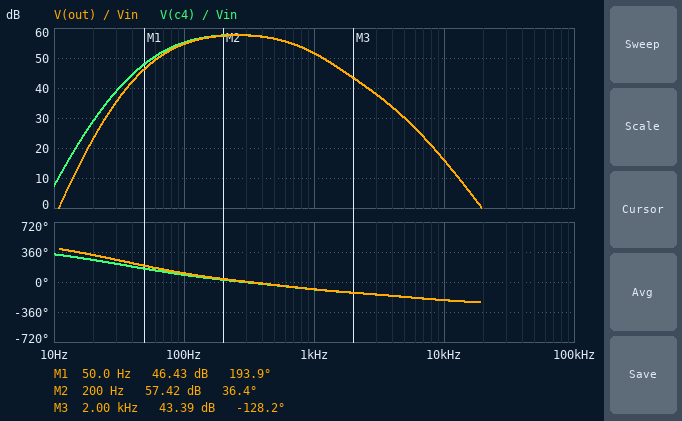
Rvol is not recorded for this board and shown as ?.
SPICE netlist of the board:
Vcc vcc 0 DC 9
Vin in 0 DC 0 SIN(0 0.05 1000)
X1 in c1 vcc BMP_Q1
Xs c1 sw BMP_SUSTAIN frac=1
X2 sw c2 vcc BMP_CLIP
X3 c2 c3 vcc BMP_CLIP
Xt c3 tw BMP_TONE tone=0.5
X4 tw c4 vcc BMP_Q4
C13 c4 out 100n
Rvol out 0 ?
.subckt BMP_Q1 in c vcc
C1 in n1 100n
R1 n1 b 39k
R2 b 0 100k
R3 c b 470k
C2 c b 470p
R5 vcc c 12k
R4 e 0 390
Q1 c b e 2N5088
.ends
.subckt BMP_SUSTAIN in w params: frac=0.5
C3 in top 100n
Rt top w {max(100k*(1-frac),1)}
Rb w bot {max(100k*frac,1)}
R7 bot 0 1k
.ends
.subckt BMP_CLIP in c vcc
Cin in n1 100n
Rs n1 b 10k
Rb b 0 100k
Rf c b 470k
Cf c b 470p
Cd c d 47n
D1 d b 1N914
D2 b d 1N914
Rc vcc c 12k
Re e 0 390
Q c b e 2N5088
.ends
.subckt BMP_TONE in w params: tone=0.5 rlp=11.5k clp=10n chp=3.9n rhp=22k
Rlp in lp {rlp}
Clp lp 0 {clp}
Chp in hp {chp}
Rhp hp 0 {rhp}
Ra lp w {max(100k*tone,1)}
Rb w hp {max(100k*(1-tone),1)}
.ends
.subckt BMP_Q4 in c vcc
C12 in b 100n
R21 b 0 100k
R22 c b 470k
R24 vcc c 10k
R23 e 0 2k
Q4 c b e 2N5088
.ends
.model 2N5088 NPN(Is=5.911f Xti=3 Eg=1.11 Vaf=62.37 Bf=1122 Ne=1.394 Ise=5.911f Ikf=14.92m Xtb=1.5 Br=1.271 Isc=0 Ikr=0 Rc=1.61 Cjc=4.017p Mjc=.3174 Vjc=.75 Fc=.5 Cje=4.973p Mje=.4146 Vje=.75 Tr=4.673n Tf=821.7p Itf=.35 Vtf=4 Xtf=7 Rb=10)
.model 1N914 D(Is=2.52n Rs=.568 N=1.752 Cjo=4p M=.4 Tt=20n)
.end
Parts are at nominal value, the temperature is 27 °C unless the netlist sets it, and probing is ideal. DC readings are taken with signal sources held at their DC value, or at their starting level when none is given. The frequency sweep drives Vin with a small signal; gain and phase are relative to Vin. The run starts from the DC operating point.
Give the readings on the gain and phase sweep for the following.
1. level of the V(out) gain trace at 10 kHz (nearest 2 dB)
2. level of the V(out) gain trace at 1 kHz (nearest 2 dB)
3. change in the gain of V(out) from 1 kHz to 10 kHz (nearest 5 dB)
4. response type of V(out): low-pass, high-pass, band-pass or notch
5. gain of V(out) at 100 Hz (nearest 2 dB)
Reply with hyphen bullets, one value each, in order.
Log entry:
- 16 dB
- 52 dB
- -35 dB
- band-pass
- 54 dB
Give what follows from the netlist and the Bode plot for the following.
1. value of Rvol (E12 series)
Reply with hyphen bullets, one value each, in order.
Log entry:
- 47 kΩ
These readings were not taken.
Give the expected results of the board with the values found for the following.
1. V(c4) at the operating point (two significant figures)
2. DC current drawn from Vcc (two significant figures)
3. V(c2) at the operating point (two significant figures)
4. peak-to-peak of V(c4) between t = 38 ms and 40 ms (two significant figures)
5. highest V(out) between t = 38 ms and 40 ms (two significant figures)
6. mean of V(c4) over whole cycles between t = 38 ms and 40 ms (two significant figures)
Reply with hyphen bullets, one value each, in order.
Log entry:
- 6.5 V
- 1.3 mA
- 4.7 V
- 1.1 V
- 530 mV
- 6.5 V
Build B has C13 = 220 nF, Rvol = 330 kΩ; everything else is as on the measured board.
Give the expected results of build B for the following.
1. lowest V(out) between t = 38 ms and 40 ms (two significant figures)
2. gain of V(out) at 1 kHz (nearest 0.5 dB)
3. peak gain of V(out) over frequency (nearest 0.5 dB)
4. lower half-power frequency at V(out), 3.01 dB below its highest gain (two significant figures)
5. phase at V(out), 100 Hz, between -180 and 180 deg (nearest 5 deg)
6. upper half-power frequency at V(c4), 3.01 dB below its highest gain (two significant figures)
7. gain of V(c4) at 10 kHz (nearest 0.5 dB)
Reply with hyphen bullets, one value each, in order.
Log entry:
- -630 mV
- 53.0 dB
- 59.0 dB
- 95 Hz
- 90 deg
- 700 Hz
- 17.0 dB
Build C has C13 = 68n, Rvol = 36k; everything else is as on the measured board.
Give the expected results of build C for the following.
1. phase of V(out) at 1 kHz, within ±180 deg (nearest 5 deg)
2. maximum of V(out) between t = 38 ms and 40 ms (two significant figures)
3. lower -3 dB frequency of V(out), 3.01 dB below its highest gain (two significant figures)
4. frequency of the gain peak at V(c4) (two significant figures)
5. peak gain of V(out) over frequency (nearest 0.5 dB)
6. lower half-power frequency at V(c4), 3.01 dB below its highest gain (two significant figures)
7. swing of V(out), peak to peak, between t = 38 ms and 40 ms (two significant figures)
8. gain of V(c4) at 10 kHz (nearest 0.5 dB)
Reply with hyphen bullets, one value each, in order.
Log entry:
- -85 deg
- 500 mV
- 110 Hz
- 240 Hz
- 57.0 dB
- 89 Hz
- 1.0 V
- 15.5 dB
